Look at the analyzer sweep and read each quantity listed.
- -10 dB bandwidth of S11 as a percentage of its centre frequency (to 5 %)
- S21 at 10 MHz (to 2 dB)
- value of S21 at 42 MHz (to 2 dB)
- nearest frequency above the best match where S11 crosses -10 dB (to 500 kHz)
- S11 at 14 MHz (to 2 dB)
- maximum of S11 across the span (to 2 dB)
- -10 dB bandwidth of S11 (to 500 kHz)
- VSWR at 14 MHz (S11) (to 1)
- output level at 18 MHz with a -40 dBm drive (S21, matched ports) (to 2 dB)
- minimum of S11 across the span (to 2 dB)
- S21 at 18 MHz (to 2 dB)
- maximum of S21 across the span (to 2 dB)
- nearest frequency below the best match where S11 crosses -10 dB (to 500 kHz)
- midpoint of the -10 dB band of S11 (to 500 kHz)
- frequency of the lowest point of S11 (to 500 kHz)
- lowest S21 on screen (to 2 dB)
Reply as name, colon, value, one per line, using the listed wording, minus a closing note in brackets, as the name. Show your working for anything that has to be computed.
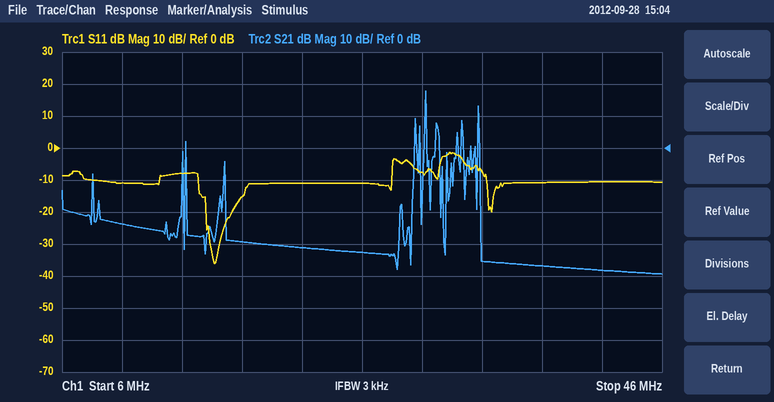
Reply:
-10 dB bandwidth of S11 as a percentage of its centre frequency: 13 MHz / 21.5 MHz ≈ 60 %
S21 at 10 MHz: -24 dB
value of S21 at 42 MHz: -38 dB
nearest frequency above the best match where S11 crosses -10 dB: 28.0 MHz
S11 at 14 MHz: -8 dB
maximum of S11 across the span: -2 dB
-10 dB bandwidth of S11: 28.0 MHz − 15.0 MHz = 13.0 MHz
VSWR at 14 MHz (S11): |Γ| = 10^(-8/20) = 0.3981; VSWR = (1 + 0.3981)/(1 − 0.3981) ≈ 2
output level at 18 MHz with a -40 dBm drive (S21, matched ports): -40 dBm + (-30 dB) = -70 dBm
minimum of S11 across the span: -36 dB
S21 at 18 MHz: -30 dB
maximum of S21 across the span: 18 dB
nearest frequency below the best match where S11 crosses -10 dB: 15.0 MHz
midpoint of the -10 dB band of S11: 21.5 MHz
frequency of the lowest point of S11: 16.0 MHz
lowest S21 on screen: -40 dB
